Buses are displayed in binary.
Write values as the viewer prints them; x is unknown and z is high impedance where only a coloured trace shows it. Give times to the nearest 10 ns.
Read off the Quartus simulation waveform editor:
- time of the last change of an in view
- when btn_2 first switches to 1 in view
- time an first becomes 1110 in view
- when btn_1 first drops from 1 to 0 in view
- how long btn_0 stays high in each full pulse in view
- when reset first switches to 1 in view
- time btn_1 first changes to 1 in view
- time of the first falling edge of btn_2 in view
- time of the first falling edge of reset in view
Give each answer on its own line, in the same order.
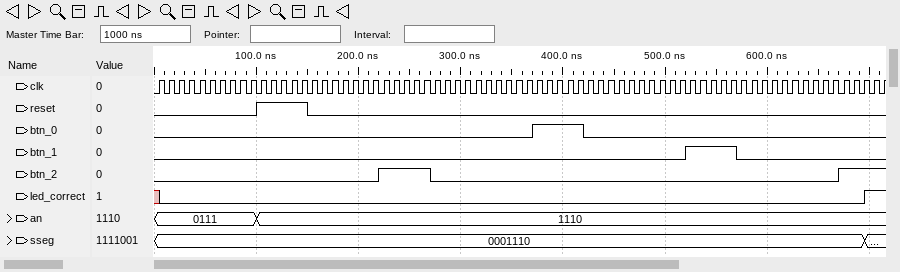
100 ns
220 ns
100 ns
570 ns
50 ns
100 ns
520 ns
270 ns
150 ns
